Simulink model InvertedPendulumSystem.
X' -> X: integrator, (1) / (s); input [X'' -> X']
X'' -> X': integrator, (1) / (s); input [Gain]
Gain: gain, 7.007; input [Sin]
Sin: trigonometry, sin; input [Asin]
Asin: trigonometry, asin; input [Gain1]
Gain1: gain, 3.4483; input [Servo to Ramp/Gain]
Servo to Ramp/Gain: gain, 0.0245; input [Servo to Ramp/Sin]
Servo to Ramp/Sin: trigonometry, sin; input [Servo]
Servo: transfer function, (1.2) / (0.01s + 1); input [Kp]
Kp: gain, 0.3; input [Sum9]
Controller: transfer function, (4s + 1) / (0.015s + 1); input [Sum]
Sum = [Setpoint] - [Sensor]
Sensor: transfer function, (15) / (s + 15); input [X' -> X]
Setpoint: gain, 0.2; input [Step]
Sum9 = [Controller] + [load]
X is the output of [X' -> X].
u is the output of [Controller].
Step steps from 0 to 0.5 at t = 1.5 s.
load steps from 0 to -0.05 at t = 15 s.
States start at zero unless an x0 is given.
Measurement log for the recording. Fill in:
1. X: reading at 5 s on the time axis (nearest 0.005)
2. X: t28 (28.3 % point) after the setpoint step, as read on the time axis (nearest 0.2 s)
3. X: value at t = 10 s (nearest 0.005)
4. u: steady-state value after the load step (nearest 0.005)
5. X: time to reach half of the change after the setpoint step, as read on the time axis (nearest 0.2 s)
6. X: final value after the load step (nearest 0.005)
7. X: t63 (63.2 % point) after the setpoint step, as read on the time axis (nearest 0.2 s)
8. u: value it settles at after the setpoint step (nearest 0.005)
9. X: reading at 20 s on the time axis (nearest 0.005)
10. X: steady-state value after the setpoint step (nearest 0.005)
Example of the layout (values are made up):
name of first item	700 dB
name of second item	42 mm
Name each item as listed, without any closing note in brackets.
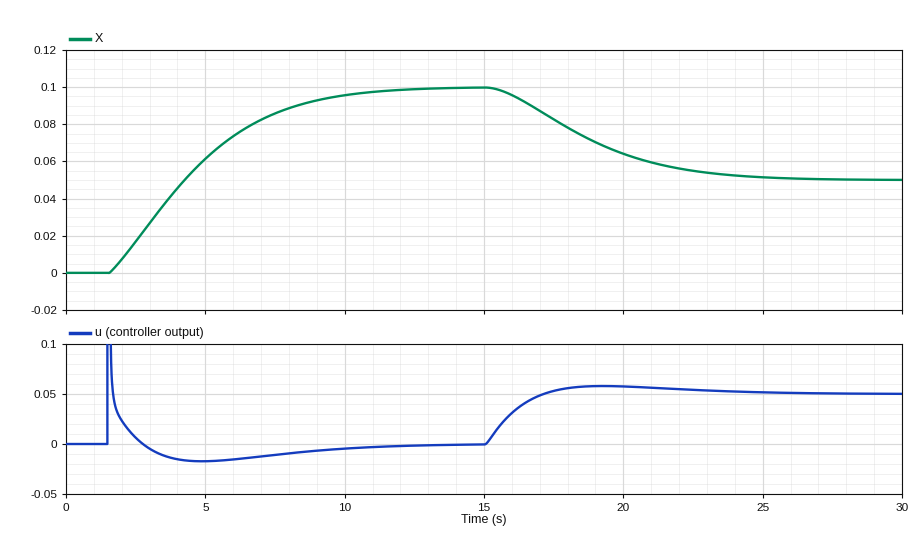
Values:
X: reading at 5 s on the time axis	0.060
X: t28 (28.3 % point) after the setpoint step, as read on the time axis	3.0 s
X: value at t = 10 s	0.095
u: steady-state value after the load step	0.050
X: time to reach half of the change after the setpoint step, as read on the time axis	4.2 s
X: final value after the load step	0.050
X: t63 (63.2 % point) after the setpoint step, as read on the time axis	5.2 s
u: value it settles at after the setpoint step	0.000
X: reading at 20 s on the time axis	0.065
X: steady-state value after the setpoint step	0.100
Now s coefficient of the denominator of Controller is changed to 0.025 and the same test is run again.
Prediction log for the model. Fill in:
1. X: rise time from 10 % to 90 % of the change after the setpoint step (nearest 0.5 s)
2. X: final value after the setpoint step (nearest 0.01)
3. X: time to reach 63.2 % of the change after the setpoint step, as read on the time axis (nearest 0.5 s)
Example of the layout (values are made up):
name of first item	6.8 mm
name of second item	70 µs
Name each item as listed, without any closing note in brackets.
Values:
X: rise time from 10 % to 90 % of the change after the setpoint step	5.0 s
X: final value after the setpoint step	0.10
X: time to reach 63.2 % of the change after the setpoint step, as read on the time axis	4.0 s
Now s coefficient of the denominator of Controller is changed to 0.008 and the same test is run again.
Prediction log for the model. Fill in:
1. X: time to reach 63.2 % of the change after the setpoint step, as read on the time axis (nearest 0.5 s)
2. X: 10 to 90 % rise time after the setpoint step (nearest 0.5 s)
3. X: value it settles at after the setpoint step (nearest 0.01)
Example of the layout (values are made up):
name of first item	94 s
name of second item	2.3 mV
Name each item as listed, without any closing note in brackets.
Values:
X: time to reach 63.2 % of the change after the setpoint step, as read on the time axis	5.5 s
X: 10 to 90 % rise time after the setpoint step	6.5 s
X: value it settles at after the setpoint step	0.10
